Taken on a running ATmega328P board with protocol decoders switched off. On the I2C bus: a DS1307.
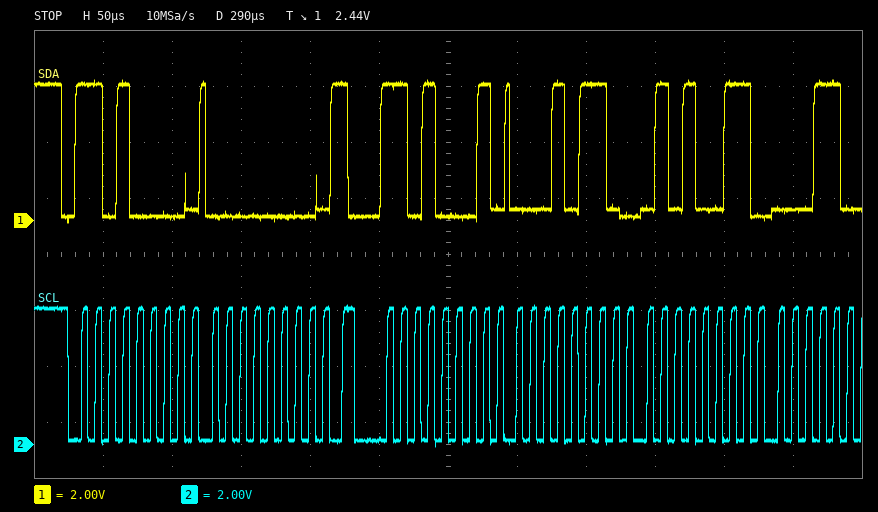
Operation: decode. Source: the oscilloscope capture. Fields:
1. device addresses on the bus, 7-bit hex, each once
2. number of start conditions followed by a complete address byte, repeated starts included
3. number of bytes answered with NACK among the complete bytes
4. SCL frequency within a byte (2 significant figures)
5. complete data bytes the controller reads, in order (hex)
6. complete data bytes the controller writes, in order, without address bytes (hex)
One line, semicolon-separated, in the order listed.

0x68; 2; 0; 100 kHz; 16 53; 00
